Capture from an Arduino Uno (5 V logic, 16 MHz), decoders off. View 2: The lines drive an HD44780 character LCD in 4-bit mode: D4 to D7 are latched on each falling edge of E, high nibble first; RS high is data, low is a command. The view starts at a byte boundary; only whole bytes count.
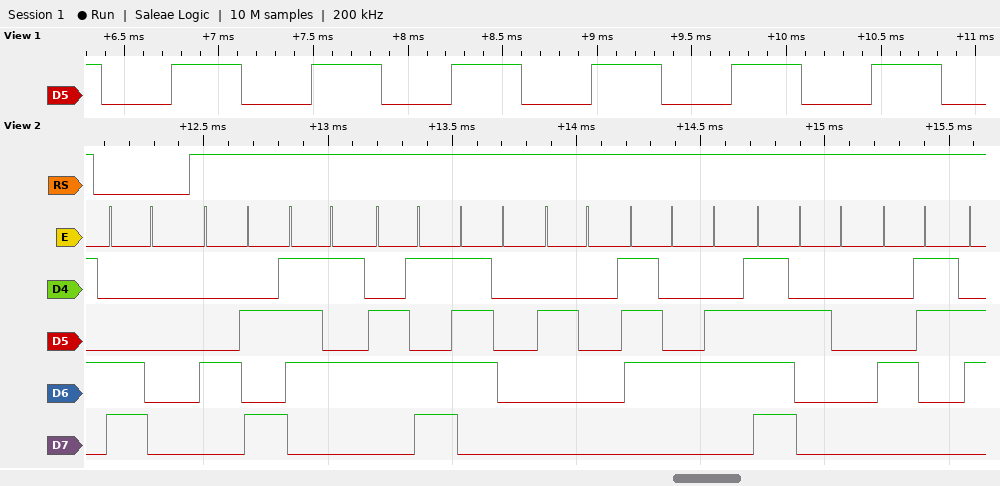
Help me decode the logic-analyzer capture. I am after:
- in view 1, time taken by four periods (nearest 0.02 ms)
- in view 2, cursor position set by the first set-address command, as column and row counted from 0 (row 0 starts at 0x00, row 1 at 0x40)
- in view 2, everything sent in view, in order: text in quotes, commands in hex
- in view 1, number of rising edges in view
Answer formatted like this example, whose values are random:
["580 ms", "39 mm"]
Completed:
["2.96 ms", "column 0, row 1", "0xC0 \"Jump to C\"", "6"]
